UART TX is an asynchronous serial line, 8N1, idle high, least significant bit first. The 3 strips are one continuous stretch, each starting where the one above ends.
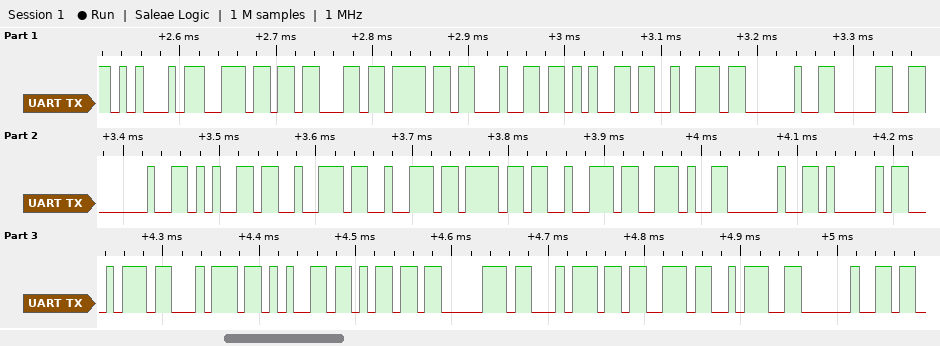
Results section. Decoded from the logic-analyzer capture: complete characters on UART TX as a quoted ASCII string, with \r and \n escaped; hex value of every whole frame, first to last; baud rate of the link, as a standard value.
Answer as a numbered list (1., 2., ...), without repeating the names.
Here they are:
1. "Encoder 0 error. Attempts: "
2. 0x45 0x6E 0x63 0x6F 0x64 0x65 0x72 0x20 0x30 0x20 0x65 0x72 0x72 0x6F 0x72 0x2E 0x20 0x41 0x74 0x74 0x65 0x6D 0x70 0x74 0x73 0x3A 0x20
3. 115200 baud
